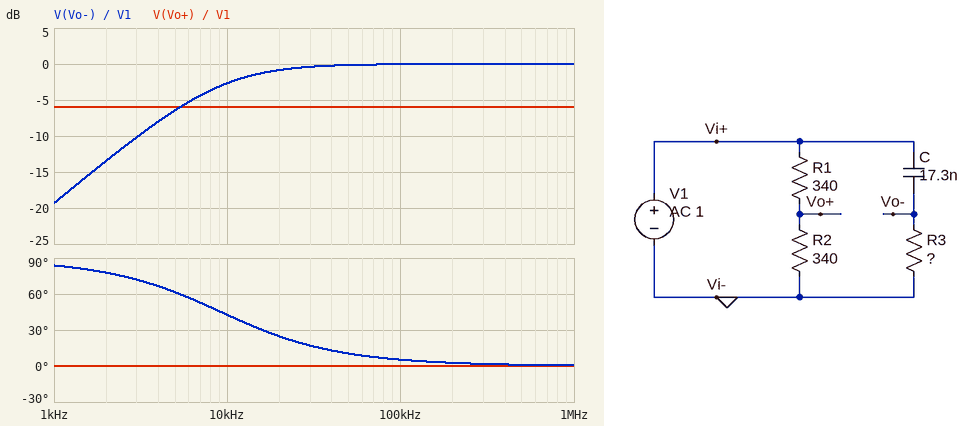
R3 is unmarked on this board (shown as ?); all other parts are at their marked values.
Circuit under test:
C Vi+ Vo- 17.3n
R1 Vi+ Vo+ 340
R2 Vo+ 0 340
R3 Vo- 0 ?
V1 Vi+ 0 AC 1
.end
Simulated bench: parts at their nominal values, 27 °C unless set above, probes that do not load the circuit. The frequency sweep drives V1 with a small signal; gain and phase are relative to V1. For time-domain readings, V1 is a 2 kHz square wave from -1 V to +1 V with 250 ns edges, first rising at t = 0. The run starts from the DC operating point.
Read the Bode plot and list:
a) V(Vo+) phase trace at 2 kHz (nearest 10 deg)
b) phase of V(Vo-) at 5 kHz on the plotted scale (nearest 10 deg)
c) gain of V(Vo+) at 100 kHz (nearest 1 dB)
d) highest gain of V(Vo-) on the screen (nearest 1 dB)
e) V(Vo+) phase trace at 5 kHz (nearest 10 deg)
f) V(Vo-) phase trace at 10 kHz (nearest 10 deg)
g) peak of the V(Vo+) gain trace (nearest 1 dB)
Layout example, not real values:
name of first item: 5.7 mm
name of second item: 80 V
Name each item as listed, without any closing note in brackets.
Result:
V(Vo+) phase trace at 2 kHz: 0 deg
phase of V(Vo-) at 5 kHz on the plotted scale: 60 deg
gain of V(Vo+) at 100 kHz: -6 dB
highest gain of V(Vo-) on the screen: 0 dB
V(Vo+) phase trace at 5 kHz: 0 deg
V(Vo-) phase trace at 10 kHz: 40 deg
peak of the V(Vo+) gain trace: -6 dB
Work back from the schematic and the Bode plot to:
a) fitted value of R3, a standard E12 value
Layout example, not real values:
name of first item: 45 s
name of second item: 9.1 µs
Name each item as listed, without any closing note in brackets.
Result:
fitted value of R3, a standard E12 value: 1 kΩ
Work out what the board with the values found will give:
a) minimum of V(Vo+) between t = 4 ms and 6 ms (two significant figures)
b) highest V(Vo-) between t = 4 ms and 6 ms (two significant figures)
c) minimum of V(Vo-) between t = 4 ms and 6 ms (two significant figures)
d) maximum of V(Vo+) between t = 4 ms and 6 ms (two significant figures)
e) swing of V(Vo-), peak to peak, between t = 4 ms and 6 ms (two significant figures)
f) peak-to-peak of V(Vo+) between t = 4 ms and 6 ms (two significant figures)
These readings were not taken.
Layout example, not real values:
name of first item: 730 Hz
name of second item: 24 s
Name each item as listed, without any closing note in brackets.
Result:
minimum of V(Vo+) between t = 4 ms and 6 ms: -500 mV
highest V(Vo-) between t = 4 ms and 6 ms: 2.0 V
minimum of V(Vo-) between t = 4 ms and 6 ms: -2.0 V
maximum of V(Vo+) between t = 4 ms and 6 ms: 500 mV
swing of V(Vo-), peak to peak, between t = 4 ms and 6 ms: 4.0 V
peak-to-peak of V(Vo+) between t = 4 ms and 6 ms: 1.0 V
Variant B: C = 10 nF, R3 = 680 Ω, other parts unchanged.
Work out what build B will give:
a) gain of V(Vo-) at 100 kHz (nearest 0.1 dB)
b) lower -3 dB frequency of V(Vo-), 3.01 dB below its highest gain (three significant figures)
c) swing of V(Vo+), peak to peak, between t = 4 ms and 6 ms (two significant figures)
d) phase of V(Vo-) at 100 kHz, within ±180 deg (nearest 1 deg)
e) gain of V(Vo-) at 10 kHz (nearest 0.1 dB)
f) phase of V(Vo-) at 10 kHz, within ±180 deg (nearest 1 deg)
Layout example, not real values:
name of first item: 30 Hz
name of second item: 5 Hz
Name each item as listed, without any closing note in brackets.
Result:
gain of V(Vo-) at 100 kHz: -0.2 dB
lower -3 dB frequency of V(Vo-), 3.01 dB below its highest gain: 23.4 kHz
swing of V(Vo+), peak to peak, between t = 4 ms and 6 ms: 1.0 V
phase of V(Vo-) at 100 kHz, within ±180 deg: 13 deg
gain of V(Vo-) at 10 kHz: -8.1 dB
phase of V(Vo-) at 10 kHz, within ±180 deg: 67 deg
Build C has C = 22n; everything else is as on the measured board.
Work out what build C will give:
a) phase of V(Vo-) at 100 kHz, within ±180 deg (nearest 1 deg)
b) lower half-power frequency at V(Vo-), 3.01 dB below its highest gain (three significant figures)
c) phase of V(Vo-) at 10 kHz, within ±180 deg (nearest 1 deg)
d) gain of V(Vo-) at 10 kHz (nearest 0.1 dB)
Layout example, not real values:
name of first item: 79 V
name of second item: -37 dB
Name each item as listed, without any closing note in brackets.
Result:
phase of V(Vo-) at 100 kHz, within ±180 deg: 4 deg
lower half-power frequency at V(Vo-), 3.01 dB below its highest gain: 7.23 kHz
phase of V(Vo-) at 10 kHz, within ±180 deg: 36 deg
gain of V(Vo-) at 10 kHz: -1.8 dB
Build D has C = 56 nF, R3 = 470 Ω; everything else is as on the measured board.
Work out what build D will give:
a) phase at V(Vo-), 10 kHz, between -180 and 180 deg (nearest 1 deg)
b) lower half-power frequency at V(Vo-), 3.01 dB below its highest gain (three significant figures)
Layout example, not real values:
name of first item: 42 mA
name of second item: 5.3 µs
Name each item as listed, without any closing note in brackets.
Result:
phase at V(Vo-), 10 kHz, between -180 and 180 deg: 31 deg
lower half-power frequency at V(Vo-), 3.01 dB below its highest gain: 6.05 kHz
